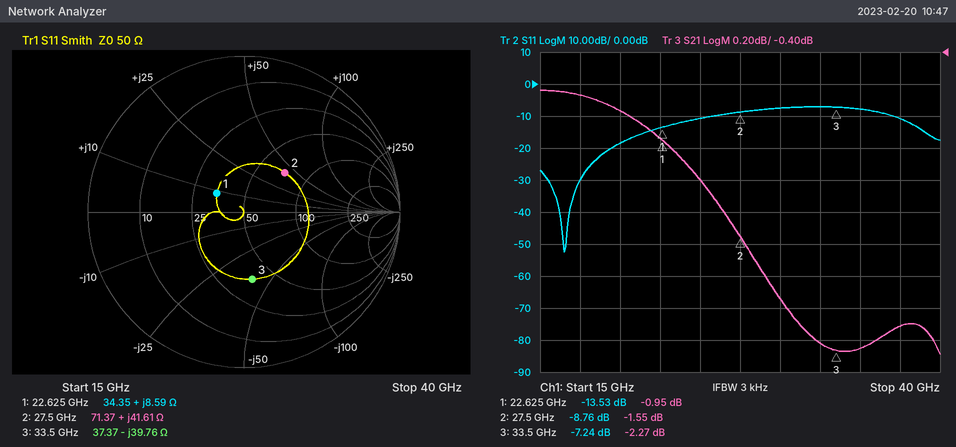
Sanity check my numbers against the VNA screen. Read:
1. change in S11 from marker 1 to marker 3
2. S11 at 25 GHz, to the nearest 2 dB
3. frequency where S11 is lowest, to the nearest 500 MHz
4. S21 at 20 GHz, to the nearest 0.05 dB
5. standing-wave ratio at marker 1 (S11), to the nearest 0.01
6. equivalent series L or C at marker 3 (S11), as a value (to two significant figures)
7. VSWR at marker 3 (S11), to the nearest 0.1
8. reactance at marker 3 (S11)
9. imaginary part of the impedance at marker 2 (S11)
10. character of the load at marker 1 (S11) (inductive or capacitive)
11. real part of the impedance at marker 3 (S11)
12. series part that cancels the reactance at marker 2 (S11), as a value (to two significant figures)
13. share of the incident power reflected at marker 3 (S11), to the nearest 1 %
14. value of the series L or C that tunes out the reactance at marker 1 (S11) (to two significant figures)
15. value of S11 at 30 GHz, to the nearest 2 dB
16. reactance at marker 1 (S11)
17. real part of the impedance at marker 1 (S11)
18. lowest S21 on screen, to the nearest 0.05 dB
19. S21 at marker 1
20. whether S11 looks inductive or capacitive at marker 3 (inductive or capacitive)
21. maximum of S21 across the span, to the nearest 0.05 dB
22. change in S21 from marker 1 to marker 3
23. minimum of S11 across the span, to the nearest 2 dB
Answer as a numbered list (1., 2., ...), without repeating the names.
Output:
1. 6.29 dB
2. -10 dB
3. 16.5 GHz
4. -0.75 dB
5. 1.53
6. 120 fF
7. 2.5
8. -39.76 Ω
9. +41.61 Ω
10. inductive
11. 37.37 Ω
12. 140 fF
13. 19 %
14. 820 fF
15. -8 dB
16. +8.59 Ω
17. 34.35 Ω
18. -2.30 dB
19. -0.95 dB
20. capacitive
21. -0.65 dB
22. -1.32 dB
23. -52 dB
